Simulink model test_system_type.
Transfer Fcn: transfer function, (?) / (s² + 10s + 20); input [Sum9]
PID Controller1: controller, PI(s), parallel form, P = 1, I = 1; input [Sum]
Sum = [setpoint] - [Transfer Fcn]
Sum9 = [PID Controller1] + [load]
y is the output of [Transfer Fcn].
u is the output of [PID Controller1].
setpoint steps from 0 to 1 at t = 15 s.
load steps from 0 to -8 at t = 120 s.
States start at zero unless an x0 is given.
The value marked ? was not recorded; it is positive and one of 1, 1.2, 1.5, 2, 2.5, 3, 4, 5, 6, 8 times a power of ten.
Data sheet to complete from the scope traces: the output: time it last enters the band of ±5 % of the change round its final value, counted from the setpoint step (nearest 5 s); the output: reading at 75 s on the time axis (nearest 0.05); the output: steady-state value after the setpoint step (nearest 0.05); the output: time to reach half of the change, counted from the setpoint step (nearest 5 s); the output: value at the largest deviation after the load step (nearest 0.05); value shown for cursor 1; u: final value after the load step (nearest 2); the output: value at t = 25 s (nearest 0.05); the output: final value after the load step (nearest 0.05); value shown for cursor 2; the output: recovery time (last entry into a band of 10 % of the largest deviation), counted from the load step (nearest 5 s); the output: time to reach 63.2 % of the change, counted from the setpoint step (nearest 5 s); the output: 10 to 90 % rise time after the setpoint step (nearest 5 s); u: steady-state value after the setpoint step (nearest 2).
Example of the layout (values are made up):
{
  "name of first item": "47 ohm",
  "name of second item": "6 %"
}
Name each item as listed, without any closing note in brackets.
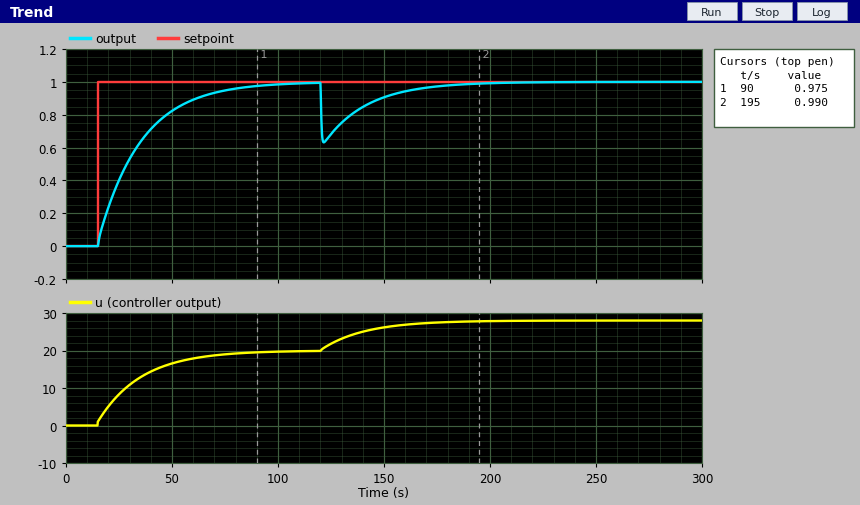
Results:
{
  "the output: time it last enters the band of ±5 % of the change round its final value, counted from the setpoint step": "60 s",
  "the output: reading at 75 s on the time axis": "0.95",
  "the output: steady-state value after the setpoint step": "1.00",
  "the output: time to reach half of the change, counted from the setpoint step": "15 s",
  "the output: value at the largest deviation after the load step": "0.65",
  "value shown for cursor 1": "0.975",
  "u: final value after the load step": "28",
  "the output: value at t = 25 s": "0.40",
  "the output: final value after the load step": "1.00",
  "value shown for cursor 2": "0.990",
  "the output: recovery time (last entry into a band of 10 % of the largest deviation), counted from the load step": "50 s",
  "the output: time to reach 63.2 % of the change, counted from the setpoint step": "20 s",
  "the output: 10 to 90 % rise time after the setpoint step": "45 s",
  "u: steady-state value after the setpoint step": "20"
}
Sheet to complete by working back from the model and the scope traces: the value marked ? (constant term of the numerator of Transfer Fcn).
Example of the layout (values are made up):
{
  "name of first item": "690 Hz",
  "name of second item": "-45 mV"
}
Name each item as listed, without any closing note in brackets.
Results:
{
  "the value marked ?": "1"
}
